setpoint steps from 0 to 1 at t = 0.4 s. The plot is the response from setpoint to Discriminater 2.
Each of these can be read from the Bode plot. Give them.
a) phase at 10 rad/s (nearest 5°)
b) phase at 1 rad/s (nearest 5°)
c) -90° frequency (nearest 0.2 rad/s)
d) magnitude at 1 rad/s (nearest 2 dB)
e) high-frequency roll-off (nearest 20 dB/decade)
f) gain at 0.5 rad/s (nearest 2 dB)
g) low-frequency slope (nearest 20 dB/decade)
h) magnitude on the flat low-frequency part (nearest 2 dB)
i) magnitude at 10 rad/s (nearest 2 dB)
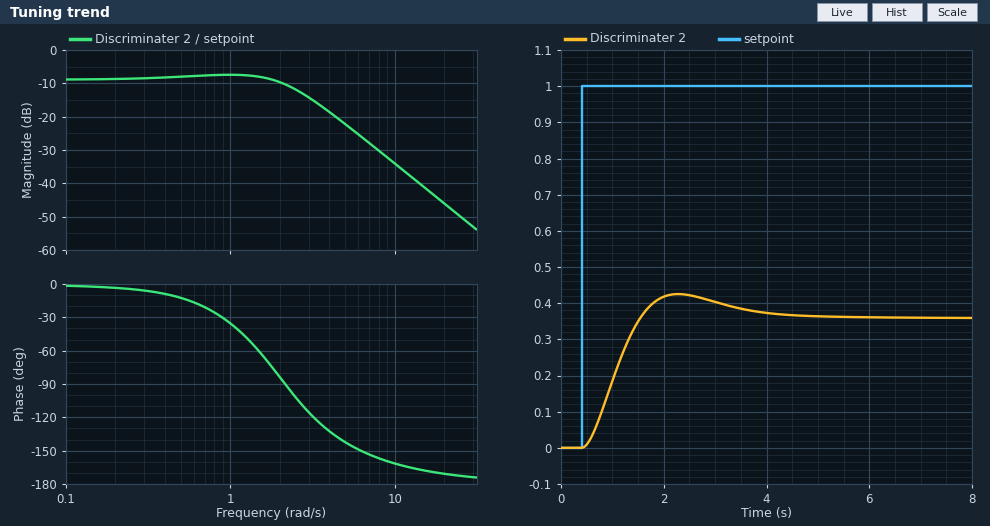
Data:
-160°
-35°
2.2 rad/s
-8 dB
-40 dB/decade
-8 dB
0 dB/decade
-8 dB
-34 dB
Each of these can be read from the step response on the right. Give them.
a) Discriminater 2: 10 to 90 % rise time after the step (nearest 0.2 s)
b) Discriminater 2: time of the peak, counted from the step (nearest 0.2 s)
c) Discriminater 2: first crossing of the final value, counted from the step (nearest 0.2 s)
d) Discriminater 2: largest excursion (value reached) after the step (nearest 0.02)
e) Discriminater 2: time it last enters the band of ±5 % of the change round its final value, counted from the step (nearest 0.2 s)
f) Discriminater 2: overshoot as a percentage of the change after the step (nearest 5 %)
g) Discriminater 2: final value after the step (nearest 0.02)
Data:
0.8 s
1.8 s
1.2 s
0.42
3.4 s
20 %
0.36
